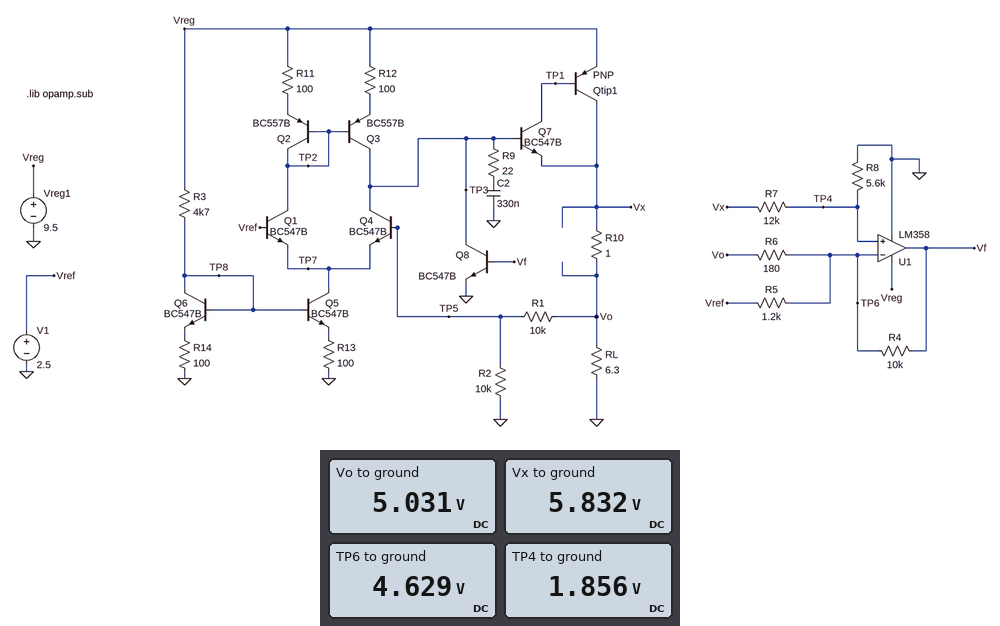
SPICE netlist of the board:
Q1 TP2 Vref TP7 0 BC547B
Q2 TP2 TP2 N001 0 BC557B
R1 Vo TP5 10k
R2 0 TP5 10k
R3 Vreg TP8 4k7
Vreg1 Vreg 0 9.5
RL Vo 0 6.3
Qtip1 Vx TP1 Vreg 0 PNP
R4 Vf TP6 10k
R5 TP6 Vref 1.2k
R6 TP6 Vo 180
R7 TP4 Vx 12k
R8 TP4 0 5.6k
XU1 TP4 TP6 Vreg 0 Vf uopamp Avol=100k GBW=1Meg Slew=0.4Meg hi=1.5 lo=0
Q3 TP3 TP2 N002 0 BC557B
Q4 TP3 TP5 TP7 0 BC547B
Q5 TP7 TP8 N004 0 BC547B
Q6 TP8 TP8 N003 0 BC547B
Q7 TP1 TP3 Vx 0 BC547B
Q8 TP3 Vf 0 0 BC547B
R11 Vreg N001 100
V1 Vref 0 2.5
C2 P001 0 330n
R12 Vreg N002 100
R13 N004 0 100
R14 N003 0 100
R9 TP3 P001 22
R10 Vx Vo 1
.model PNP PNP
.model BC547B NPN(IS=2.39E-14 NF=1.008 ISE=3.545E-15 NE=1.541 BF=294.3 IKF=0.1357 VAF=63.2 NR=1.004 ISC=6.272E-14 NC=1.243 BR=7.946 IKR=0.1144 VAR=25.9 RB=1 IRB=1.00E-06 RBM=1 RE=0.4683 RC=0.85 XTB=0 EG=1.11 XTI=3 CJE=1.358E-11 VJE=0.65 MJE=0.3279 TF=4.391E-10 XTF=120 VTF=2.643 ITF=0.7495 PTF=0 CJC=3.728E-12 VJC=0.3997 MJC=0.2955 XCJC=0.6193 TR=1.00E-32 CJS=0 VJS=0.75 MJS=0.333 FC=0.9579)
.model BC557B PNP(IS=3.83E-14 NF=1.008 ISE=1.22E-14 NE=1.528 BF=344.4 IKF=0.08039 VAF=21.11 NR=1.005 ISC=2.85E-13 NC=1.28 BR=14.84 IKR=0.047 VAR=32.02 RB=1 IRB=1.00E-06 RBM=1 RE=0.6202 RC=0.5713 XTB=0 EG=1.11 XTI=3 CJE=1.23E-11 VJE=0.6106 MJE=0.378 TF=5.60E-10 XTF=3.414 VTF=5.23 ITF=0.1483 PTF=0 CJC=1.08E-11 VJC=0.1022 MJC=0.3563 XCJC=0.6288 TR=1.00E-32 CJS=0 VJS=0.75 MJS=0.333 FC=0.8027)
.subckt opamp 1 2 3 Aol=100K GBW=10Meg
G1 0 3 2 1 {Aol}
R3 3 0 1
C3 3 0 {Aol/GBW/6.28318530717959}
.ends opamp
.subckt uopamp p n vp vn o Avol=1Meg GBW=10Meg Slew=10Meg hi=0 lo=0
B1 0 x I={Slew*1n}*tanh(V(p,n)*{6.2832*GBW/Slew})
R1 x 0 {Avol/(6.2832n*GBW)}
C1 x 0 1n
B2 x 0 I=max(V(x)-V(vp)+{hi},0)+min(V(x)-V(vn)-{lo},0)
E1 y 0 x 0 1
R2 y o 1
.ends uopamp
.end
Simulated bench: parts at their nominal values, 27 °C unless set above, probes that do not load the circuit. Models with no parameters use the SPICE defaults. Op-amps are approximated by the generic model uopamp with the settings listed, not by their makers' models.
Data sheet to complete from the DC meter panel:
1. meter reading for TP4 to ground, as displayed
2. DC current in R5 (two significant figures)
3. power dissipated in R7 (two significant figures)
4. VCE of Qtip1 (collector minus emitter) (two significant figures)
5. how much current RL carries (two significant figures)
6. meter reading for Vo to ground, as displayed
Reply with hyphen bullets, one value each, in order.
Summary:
- 1.856 V
- 1.8 mA
- 1.3 mW
- -3.7 V
- 800 mA
- 5.031 V
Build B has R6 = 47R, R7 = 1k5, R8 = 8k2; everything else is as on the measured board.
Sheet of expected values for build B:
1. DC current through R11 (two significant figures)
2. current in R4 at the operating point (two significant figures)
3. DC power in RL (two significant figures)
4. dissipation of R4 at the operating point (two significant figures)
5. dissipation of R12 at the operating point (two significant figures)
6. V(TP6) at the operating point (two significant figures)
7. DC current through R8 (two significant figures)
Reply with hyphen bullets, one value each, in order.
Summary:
- 1.8 mA
- 370 µA
- 3.1 W
- 1.3 mW
- 340 µW
- 4.3 V
- 530 µA
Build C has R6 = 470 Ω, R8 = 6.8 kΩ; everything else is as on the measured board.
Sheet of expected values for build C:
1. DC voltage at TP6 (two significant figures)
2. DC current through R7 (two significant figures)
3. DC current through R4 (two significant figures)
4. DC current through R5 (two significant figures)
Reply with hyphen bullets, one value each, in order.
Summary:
- 4.2 V
- 310 µA
- 420 µA
- 1.4 mA
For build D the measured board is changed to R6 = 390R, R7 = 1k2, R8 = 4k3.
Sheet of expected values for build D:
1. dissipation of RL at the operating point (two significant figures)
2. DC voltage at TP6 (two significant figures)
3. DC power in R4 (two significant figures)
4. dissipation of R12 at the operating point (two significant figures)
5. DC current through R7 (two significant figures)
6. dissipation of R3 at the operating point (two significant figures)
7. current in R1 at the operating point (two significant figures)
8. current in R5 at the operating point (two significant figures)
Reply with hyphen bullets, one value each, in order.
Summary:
- 2.0 W
- 3.2 V
- 660 µW
- 350 µW
- 750 µA
- 16 mW
- 180 µA
- 600 µA
